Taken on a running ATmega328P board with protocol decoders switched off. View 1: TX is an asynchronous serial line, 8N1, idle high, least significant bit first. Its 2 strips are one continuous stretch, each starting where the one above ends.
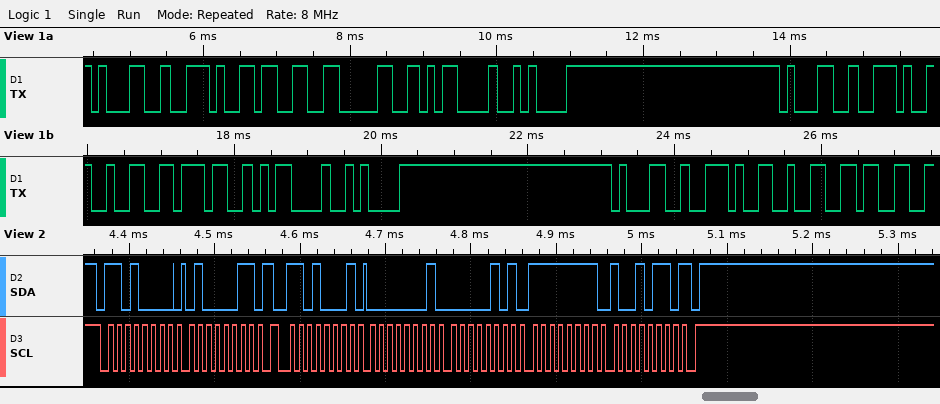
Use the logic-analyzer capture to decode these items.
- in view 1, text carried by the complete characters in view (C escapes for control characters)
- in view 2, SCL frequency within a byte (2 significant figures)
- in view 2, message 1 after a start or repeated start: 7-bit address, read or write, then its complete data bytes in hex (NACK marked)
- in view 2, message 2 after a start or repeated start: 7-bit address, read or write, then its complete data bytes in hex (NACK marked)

"1.30\r\n1.27\r\n1.23"
100 kHz
0x68 write: 43
0x68 read: 01 05 FF 96 NACK
